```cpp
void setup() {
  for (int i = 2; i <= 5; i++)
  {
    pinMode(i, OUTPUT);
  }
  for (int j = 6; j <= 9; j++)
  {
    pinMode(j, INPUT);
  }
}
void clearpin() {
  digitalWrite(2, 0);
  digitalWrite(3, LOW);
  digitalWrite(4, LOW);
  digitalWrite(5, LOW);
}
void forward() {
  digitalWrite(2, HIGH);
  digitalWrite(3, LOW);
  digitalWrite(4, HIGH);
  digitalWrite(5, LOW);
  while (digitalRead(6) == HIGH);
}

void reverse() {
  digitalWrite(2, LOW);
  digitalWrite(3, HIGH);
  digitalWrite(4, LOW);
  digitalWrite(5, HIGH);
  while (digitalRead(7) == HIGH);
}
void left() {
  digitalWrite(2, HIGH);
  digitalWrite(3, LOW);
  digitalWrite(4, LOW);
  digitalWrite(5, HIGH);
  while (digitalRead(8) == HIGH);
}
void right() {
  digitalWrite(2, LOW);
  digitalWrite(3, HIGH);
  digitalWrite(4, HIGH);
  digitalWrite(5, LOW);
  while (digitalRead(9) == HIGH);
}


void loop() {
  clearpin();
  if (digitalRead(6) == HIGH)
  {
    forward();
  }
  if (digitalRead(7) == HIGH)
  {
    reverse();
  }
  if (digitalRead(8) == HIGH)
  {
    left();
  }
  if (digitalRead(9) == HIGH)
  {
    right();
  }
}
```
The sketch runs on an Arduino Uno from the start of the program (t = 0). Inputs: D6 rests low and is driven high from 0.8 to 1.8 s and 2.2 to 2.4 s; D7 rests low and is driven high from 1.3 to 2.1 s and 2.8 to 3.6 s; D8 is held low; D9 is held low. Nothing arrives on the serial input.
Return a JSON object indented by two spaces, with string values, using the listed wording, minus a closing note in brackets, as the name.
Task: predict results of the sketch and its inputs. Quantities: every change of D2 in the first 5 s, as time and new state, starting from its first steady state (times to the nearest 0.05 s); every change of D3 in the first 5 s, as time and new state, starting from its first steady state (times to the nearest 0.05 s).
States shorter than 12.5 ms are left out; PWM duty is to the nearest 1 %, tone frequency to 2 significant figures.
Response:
{
  "every change of D2 in the first 5 s, as time and new state, starting from its first steady state": "0 s low; 0.8 s high; 1.8 s low; 2.2 s high; 2.4 s low",
  "every change of D3 in the first 5 s, as time and new state, starting from its first steady state": "0 s low; 1.8 s high; 2.1 s low; 2.8 s high; 3.6 s low"
}
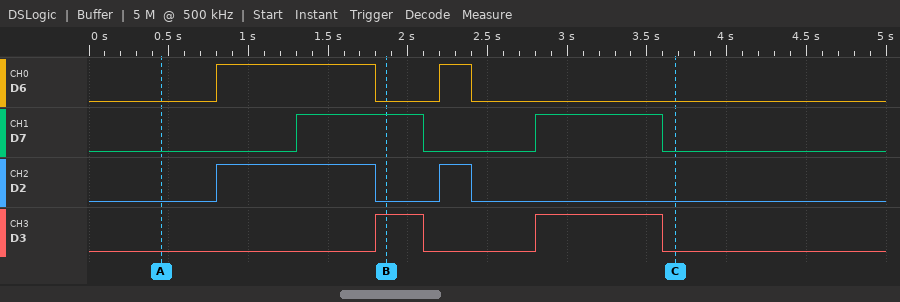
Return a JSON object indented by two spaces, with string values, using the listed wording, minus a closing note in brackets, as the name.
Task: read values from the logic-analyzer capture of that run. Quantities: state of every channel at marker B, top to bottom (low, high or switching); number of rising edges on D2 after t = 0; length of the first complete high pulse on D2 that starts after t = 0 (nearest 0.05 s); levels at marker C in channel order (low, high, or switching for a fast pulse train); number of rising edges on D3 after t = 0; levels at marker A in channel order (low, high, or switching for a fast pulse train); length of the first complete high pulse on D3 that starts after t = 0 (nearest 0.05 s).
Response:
{
  "state of every channel at marker B, top to bottom": "D6 low, D7 high, D2 low, D3 high",
  "number of rising edges on D2 after t = 0": "2",
  "length of the first complete high pulse on D2 that starts after t = 0": "1.00 s",
  "levels at marker C in channel order": "D6 low, D7 low, D2 low, D3 low",
  "number of rising edges on D3 after t = 0": "2",
  "levels at marker A in channel order": "D6 low, D7 low, D2 low, D3 low",
  "length of the first complete high pulse on D3 that starts after t = 0": "0.30 s"
}
